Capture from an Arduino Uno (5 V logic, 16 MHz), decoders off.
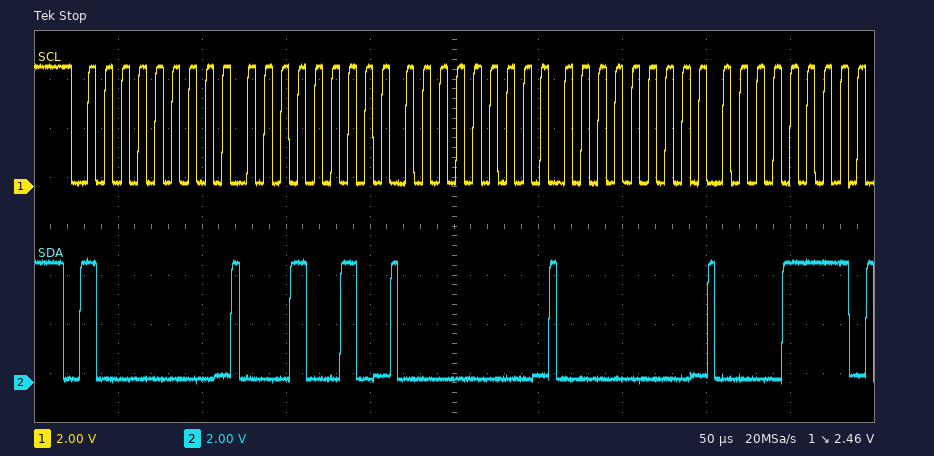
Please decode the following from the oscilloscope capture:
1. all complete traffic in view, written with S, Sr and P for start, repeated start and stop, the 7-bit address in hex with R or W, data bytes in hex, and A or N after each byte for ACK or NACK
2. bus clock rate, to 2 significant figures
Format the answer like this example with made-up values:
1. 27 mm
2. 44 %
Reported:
1. S 40W A 12 A 00 A 00 A 0F A
2. 100 kHz
